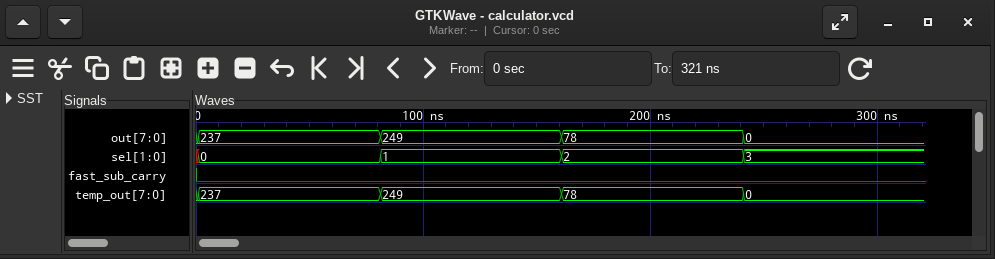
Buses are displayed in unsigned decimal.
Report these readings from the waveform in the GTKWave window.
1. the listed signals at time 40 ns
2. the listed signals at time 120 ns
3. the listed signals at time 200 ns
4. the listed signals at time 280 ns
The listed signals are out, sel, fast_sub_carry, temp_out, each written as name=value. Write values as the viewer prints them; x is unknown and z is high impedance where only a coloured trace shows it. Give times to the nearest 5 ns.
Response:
out=237, sel=0, fast_sub_carry=0, temp_out=237
out=249, sel=1, fast_sub_carry=0, temp_out=249
out=78, sel=2, fast_sub_carry=0, temp_out=78
out=0, sel=3, fast_sub_carry=0, temp_out=0
